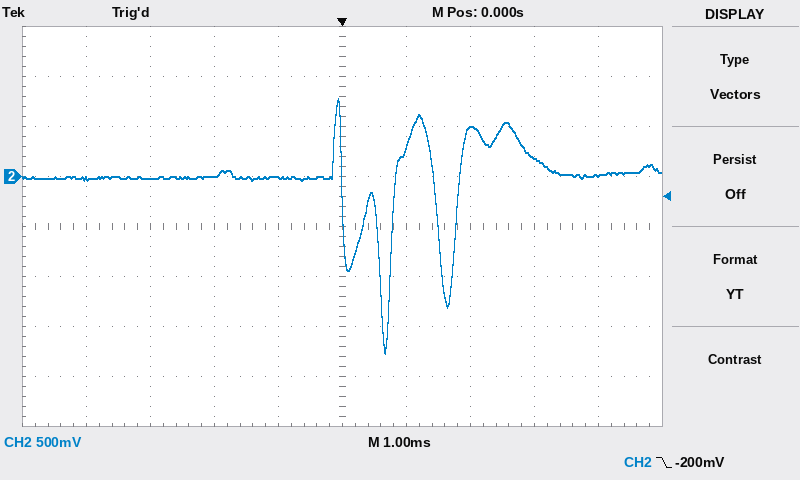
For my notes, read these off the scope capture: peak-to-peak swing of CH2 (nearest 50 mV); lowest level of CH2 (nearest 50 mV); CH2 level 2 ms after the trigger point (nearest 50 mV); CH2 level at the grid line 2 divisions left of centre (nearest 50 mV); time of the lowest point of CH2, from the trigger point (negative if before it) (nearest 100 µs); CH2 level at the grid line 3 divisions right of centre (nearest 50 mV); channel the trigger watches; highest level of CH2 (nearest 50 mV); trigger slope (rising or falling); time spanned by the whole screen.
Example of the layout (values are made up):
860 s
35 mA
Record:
2.55 V
-1.75 V
500 mV
0 mV
+700 µs
200 mV
CH2
800 mV
falling
10 ms
